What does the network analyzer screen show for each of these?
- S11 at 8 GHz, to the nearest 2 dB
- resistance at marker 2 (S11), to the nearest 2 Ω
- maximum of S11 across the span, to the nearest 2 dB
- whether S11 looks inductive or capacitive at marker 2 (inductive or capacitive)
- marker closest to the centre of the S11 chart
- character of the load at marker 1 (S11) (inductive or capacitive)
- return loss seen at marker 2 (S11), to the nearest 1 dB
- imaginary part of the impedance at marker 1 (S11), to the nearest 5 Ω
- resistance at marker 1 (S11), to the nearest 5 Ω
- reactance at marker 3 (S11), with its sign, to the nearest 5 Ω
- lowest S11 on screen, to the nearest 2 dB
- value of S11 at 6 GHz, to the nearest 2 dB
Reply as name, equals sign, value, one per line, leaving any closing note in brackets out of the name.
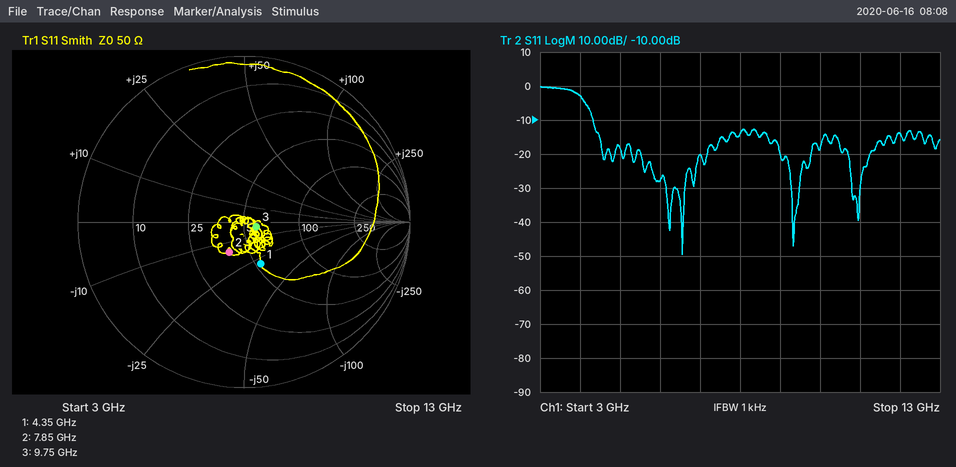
S11 at 8 GHz, to the nearest 2 dB = -14 dB
resistance at marker 2 (S11), to the nearest 2 Ω = 40 Ω
maximum of S11 across the span, to the nearest 2 dB = 0 dB
whether S11 looks inductive or capacitive at marker 2 = capacitive
marker closest to the centre of the S11 chart = marker 3
character of the load at marker 1 (S11) = capacitive
return loss seen at marker 2 (S11), to the nearest 1 dB = 14 dB
imaginary part of the impedance at marker 1 (S11), to the nearest 5 Ω = -30 Ω
resistance at marker 1 (S11), to the nearest 5 Ω = 55 Ω
reactance at marker 3 (S11), with its sign, to the nearest 5 Ω = -5 Ω
lowest S11 on screen, to the nearest 2 dB = -50 dB
value of S11 at 6 GHz, to the nearest 2 dB = -28 dB
